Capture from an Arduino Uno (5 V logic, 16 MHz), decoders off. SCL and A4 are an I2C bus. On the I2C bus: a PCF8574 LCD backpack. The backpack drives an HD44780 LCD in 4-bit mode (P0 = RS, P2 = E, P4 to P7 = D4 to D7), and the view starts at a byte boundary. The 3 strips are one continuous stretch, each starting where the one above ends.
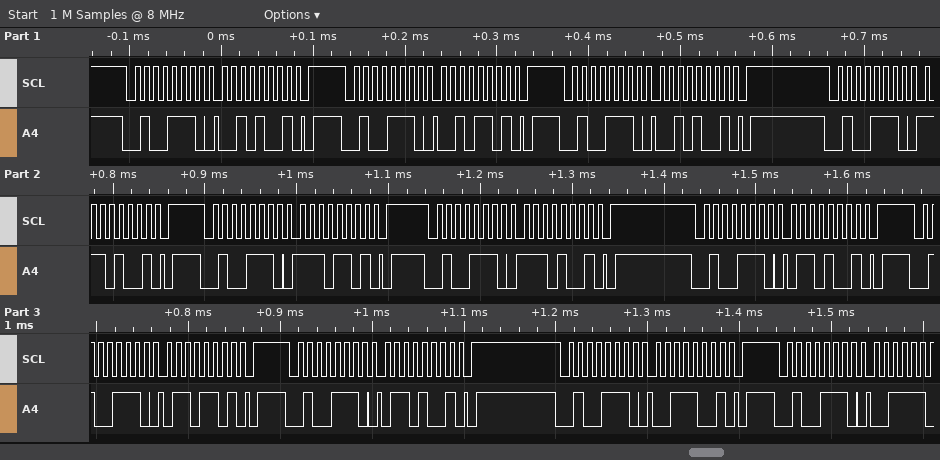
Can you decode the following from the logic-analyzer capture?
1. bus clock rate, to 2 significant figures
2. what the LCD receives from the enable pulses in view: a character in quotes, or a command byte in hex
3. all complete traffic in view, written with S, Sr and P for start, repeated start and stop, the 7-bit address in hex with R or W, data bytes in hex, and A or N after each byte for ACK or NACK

100 kHz
'.'
S 27W A 29 A P S 27W A 2D A P S 27W A 29 A P S 27W A E9 A P S 27W A ED A P S 27W A E9 A P S 27W A 69 A P S 27W A 6D A P S 27W A 69 A P S 27W A 39 A P S 27W A
